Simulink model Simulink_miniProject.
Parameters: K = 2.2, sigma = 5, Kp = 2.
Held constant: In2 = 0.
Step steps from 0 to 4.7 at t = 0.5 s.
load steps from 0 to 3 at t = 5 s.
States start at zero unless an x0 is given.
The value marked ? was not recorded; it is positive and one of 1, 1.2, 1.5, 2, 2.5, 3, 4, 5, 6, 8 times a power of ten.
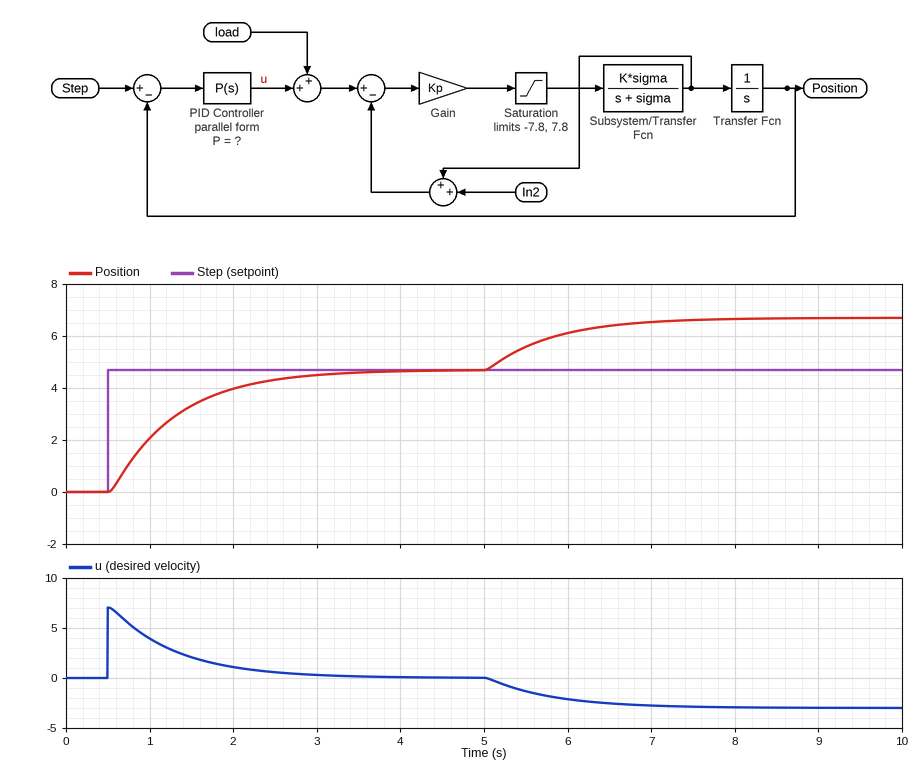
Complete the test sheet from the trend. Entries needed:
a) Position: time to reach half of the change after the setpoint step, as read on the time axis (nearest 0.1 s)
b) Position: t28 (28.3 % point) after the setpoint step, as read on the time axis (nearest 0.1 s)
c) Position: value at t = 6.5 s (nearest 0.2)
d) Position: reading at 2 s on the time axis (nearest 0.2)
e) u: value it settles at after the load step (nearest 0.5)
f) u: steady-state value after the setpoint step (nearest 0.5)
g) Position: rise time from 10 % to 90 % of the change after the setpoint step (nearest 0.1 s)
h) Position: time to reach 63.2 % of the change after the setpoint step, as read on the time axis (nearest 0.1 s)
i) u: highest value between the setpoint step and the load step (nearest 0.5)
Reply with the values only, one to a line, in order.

1.1 s
0.8 s
6.4
4.0
-3.0
0.0
1.7 s
1.3 s
7.0
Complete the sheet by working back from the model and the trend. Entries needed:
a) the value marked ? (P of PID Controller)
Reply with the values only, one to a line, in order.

1.5
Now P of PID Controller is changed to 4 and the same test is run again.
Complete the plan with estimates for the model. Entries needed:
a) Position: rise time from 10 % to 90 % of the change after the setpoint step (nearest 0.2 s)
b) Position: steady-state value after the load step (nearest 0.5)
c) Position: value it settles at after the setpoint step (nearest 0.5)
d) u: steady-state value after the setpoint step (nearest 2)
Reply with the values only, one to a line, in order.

0.6 s
5.5
4.5
0
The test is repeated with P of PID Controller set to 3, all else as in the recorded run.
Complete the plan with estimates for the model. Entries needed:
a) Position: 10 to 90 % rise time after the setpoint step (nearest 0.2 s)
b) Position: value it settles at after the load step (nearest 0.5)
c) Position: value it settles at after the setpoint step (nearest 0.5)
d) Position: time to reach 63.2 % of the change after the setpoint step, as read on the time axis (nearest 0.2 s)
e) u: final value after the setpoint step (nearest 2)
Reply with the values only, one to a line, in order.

0.8 s
5.5
4.5
1.0 s
0
